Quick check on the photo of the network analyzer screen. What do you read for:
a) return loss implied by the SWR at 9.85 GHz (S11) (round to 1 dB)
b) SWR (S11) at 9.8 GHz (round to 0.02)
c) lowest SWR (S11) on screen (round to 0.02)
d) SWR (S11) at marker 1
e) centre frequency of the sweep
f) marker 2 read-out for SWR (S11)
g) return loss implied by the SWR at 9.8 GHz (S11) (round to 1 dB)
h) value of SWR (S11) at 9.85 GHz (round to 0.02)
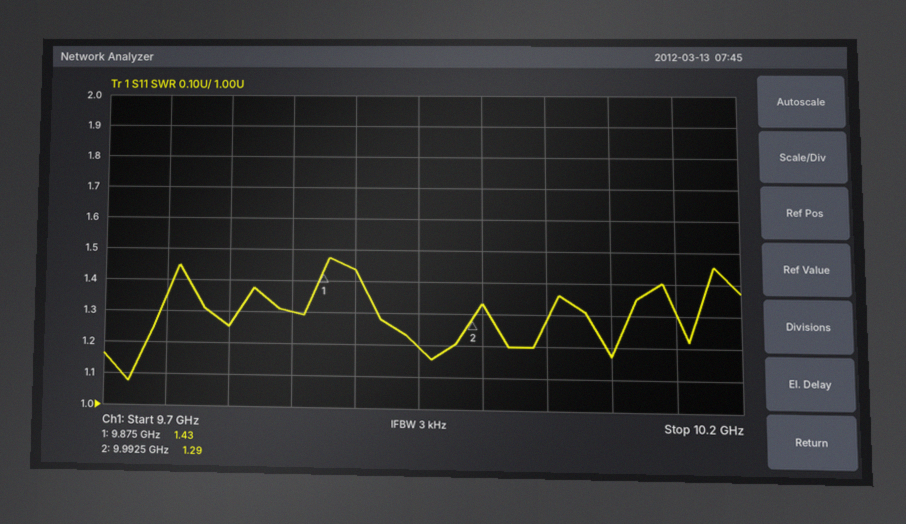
18 dB
1.26
1.08
1.43
9.95 GHz
1.29
19 dB
1.30
